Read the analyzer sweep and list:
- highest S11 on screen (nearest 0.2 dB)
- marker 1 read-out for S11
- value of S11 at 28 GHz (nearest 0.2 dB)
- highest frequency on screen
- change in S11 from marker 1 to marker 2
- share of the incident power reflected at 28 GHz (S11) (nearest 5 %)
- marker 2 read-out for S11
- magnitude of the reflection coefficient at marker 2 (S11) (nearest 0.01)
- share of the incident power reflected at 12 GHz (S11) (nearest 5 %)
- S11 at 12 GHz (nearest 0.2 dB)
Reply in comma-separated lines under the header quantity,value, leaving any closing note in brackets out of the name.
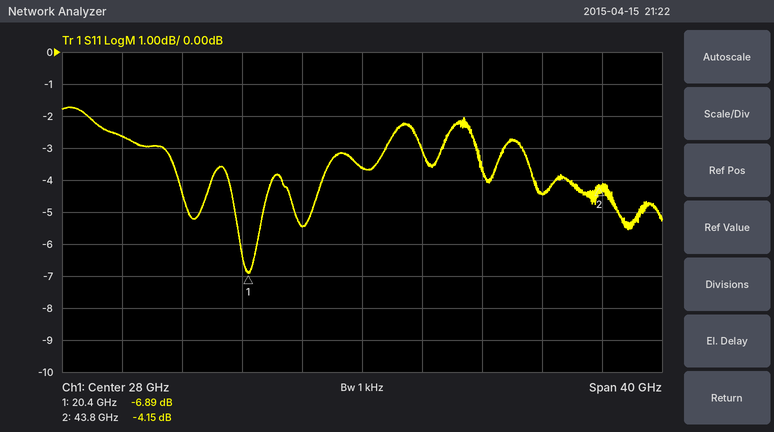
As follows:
quantity,value
highest S11 on screen,-1.8 dB
marker 1 read-out for S11,-6.89 dB
value of S11 at 28 GHz,-3.6 dB
highest frequency on screen,48 GHz
change in S11 from marker 1 to marker 2,2.74 dB
share of the incident power reflected at 28 GHz (S11),45 %
marker 2 read-out for S11,-4.15 dB
magnitude of the reflection coefficient at marker 2 (S11),0.62
share of the incident power reflected at 12 GHz (S11),55 %
S11 at 12 GHz,-2.6 dB
